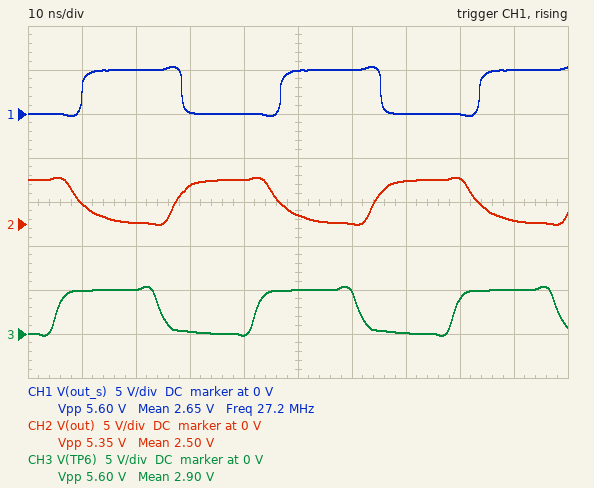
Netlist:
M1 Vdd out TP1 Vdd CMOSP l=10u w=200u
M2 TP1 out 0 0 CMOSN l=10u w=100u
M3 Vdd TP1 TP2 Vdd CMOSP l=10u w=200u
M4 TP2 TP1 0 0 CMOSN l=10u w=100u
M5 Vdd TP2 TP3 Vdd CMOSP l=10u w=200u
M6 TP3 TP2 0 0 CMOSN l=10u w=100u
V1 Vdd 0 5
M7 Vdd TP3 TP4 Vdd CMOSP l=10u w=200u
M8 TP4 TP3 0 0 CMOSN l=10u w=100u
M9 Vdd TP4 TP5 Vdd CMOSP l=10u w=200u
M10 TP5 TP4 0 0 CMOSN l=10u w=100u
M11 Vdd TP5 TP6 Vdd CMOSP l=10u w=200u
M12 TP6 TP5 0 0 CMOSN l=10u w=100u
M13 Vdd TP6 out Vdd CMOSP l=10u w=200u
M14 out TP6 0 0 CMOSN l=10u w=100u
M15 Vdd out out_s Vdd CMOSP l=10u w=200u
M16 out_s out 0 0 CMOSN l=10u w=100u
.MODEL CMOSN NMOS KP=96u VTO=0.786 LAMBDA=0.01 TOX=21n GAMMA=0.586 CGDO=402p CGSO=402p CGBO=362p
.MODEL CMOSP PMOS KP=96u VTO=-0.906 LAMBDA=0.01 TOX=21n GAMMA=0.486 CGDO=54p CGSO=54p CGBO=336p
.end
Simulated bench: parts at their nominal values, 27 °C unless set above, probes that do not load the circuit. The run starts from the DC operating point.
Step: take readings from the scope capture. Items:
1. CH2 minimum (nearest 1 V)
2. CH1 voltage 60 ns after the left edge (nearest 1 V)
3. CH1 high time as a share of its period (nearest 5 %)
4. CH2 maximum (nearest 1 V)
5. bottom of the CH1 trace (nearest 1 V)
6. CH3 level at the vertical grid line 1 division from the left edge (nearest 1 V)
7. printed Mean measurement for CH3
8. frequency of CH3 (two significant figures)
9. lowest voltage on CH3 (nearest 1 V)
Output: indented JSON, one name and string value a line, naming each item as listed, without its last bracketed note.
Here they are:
{
  "CH2 minimum": "0 V",
  "CH1 voltage 60 ns after the left edge": "5 V",
  "CH1 high time as a share of its period": "50 %",
  "CH2 maximum": "5 V",
  "bottom of the CH1 trace": "0 V",
  "CH3 level at the vertical grid line 1 division from the left edge": "5 V",
  "printed Mean measurement for CH3": "2.90 V",
  "frequency of CH3": "27 MHz",
  "lowest voltage on CH3": "0 V"
}
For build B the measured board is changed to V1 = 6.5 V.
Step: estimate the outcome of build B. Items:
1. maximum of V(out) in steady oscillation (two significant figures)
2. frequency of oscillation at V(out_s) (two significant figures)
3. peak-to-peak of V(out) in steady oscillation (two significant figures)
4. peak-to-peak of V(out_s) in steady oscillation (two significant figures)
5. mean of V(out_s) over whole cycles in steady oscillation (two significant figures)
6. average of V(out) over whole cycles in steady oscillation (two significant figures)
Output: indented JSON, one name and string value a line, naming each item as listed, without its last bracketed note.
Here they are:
{
  "maximum of V(out) in steady oscillation": "6.8 V",
  "frequency of oscillation at V(out_s)": "39 MHz",
  "peak-to-peak of V(out) in steady oscillation": "6.9 V",
  "peak-to-peak of V(out_s) in steady oscillation": "7.3 V",
  "mean of V(out_s) over whole cycles in steady oscillation": "3.3 V",
  "average of V(out) over whole cycles in steady oscillation": "3.5 V"
}
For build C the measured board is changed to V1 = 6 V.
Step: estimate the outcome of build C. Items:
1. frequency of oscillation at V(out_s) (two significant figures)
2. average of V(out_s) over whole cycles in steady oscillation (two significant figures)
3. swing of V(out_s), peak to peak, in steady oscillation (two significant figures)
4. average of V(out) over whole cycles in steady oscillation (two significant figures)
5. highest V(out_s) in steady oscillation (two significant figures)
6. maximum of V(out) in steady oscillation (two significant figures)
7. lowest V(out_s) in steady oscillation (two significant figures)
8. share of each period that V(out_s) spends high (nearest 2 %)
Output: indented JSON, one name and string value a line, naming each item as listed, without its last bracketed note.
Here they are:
{
  "frequency of oscillation at V(out_s)": "35 MHz",
  "average of V(out_s) over whole cycles in steady oscillation": "3.0 V",
  "swing of V(out_s), peak to peak, in steady oscillation": "6.7 V",
  "average of V(out) over whole cycles in steady oscillation": "3.2 V",
  "highest V(out_s) in steady oscillation": "6.4 V",
  "maximum of V(out) in steady oscillation": "6.3 V",
  "lowest V(out_s) in steady oscillation": "-300 mV",
  "share of each period that V(out_s) spends high": "50 %"
}
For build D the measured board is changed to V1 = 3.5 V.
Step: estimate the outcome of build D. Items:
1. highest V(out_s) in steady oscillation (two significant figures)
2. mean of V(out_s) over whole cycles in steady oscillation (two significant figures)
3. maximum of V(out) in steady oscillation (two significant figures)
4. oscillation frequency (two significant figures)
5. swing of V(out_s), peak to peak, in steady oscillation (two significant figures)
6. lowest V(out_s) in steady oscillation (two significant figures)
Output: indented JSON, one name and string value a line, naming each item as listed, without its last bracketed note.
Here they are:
{
  "highest V(out_s) in steady oscillation": "3.8 V",
  "mean of V(out_s) over whole cycles in steady oscillation": "1.8 V",
  "maximum of V(out) in steady oscillation": "3.7 V",
  "oscillation frequency": "16 MHz",
  "swing of V(out_s), peak to peak, in steady oscillation": "4.0 V",
  "lowest V(out_s) in steady oscillation": "-200 mV"
}
